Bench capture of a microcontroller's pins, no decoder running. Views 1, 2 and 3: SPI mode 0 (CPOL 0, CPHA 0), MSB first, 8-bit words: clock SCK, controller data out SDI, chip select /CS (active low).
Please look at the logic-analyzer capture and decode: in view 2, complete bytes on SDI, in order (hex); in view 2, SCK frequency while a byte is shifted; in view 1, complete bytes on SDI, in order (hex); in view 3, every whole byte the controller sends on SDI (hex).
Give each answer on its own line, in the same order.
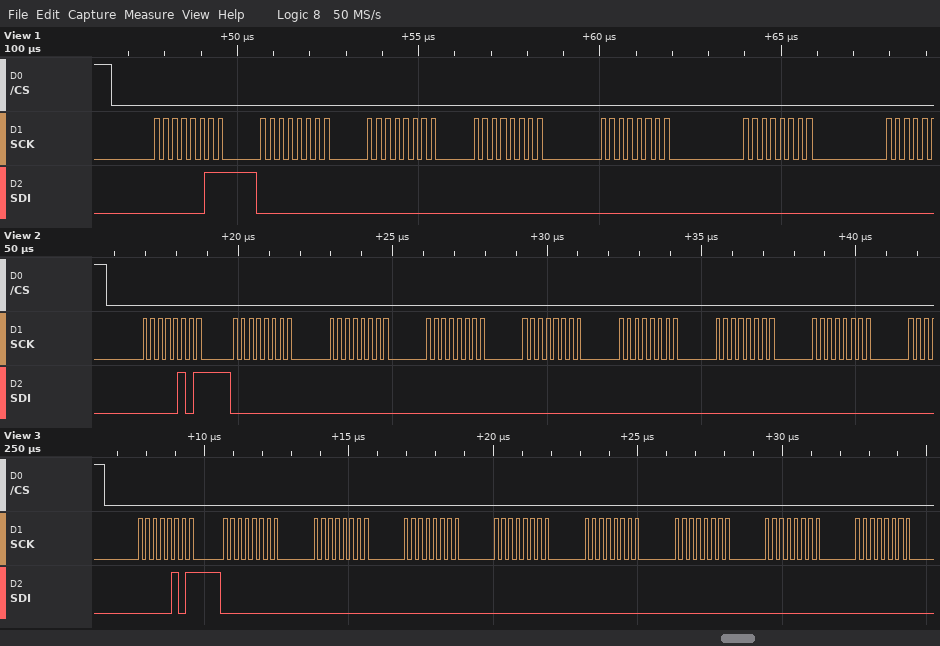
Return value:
05 00 00 00 00 00 00 00
4 MHz
0x03 0x00 0x00 0x00 0x00 0x00
05 00 00 00 00 00 00 00 00
